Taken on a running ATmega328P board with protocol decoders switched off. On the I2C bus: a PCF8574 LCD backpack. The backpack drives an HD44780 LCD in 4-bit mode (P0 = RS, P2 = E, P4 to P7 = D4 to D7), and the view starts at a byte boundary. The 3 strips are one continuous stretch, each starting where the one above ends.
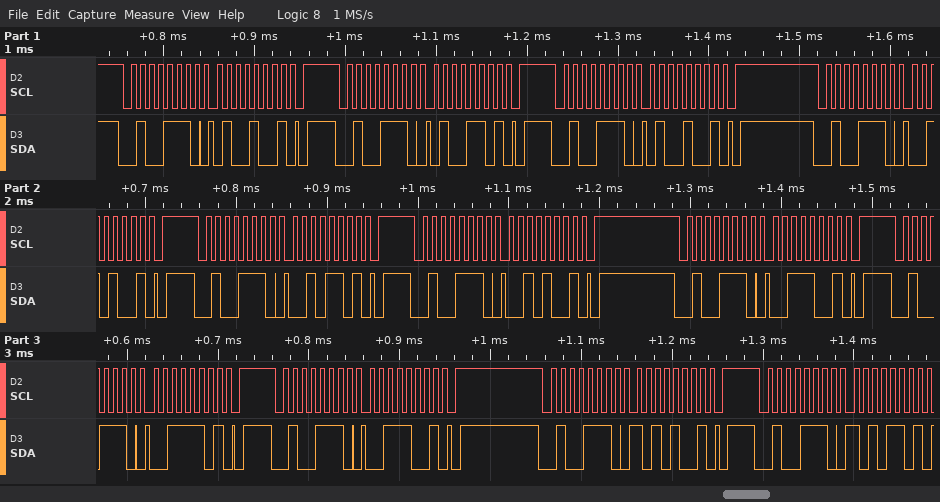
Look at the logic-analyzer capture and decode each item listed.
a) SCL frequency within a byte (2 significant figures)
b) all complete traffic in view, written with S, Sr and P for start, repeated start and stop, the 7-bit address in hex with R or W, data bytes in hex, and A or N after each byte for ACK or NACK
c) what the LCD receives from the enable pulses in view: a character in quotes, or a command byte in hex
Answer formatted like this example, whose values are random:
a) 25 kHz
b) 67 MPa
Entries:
a) 100 kHz
b) S 27W A 49 A P S 27W A 4D A P S 27W A 49 A P S 27W A 29 A P S 27W A 2D A P S 27W A 29 A P S 27W A 39 A P S 27W A 3D A P S 27W A 39 A P S 27W A A9 A P S 27W A AD A
c) 'B'
